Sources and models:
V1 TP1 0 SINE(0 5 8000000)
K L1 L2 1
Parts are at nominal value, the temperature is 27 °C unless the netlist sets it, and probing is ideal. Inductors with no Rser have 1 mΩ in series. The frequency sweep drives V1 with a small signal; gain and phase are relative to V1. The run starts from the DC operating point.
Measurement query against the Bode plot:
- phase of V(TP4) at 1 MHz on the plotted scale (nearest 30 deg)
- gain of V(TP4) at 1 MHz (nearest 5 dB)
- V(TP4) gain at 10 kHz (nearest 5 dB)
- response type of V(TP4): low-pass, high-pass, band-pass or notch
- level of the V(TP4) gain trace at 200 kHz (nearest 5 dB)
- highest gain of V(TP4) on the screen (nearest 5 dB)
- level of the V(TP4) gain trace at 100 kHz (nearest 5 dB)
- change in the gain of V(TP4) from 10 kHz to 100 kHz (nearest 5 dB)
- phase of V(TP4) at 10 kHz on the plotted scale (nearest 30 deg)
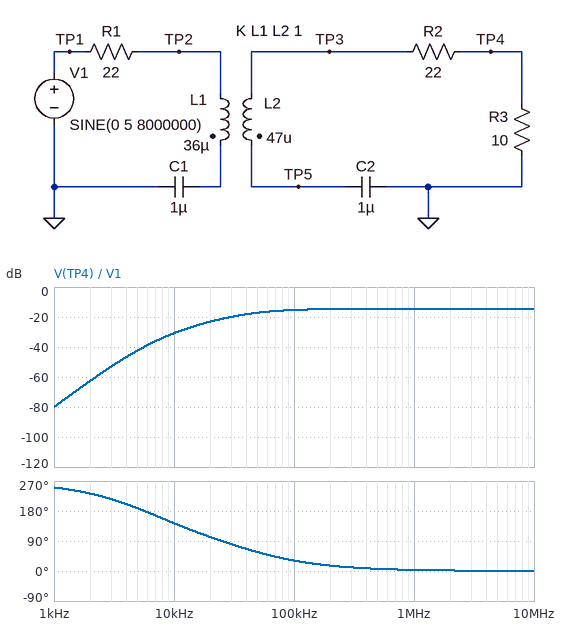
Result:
0 deg
-15 dB
-30 dB
high-pass
-15 dB
-15 dB
-15 dB
15 dB
150 deg
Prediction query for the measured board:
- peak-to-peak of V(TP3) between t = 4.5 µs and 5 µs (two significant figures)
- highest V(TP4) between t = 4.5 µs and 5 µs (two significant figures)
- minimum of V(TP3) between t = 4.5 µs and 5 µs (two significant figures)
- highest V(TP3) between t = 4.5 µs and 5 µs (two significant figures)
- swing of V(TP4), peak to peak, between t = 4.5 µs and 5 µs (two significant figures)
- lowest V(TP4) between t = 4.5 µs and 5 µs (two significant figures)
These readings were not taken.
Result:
6.0 V
940 mV
-3.0 V
3.0 V
1.9 V
-940 mV
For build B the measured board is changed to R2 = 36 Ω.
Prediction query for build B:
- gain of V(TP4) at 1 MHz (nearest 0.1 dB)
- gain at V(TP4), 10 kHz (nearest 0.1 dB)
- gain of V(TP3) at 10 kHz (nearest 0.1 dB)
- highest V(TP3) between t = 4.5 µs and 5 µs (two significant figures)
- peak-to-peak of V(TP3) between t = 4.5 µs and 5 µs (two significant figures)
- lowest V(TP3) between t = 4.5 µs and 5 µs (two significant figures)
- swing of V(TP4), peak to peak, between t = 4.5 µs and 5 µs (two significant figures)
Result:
-16.3 dB
-33.6 dB
-20.4 dB
3.5 V
7.0 V
-3.5 V
1.5 V
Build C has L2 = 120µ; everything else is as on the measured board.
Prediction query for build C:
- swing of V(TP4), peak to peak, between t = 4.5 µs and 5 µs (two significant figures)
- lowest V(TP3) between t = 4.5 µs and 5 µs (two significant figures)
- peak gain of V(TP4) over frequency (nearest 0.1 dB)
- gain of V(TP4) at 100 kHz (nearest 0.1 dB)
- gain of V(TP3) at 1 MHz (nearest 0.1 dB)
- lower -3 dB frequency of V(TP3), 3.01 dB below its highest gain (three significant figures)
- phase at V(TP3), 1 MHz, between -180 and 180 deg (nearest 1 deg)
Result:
1.7 V
-2.8 V
-15.2 dB
-15.5 dB
-5.1 dB
25.8 kHz
2 deg
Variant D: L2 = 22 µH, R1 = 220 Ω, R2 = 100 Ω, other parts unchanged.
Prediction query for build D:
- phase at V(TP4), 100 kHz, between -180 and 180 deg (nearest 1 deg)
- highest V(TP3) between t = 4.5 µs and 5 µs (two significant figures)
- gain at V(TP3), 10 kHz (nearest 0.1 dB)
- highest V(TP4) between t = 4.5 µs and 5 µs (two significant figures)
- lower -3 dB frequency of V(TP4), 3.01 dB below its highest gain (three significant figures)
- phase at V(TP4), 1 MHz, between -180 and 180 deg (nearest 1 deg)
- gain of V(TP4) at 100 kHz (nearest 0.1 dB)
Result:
78 deg
1.8 V
-42.0 dB
160 mV
437 kHz
24 deg
-42.9 dB
